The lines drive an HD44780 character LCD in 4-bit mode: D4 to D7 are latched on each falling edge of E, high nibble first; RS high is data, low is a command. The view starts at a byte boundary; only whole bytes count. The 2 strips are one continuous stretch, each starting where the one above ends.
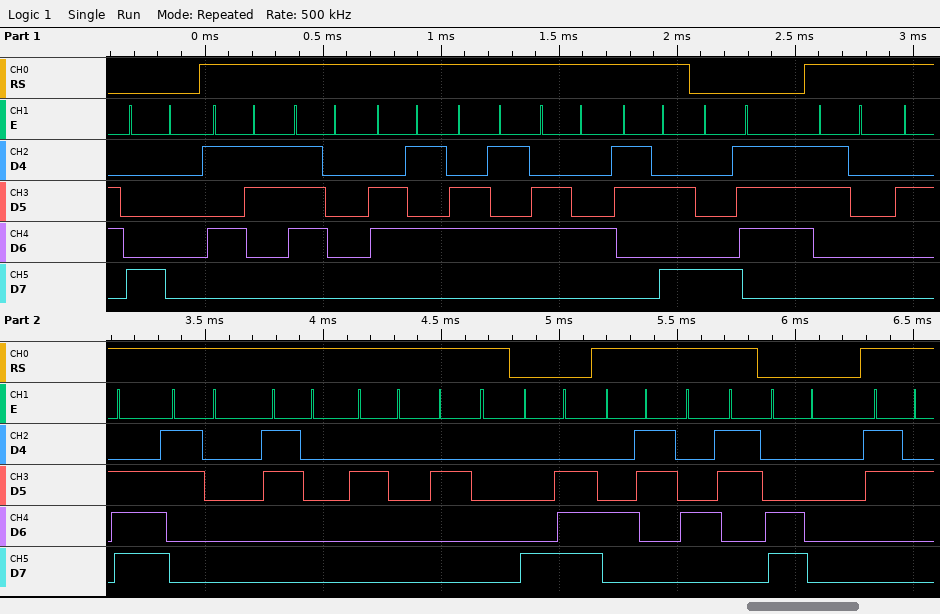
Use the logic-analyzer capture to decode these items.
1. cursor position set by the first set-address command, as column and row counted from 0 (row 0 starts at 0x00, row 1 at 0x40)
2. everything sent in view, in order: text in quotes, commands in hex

column 0, row 0
0x80 "Speed:" 0x87 "0.00  " 0x8E "CC" 0xC0 "2"
